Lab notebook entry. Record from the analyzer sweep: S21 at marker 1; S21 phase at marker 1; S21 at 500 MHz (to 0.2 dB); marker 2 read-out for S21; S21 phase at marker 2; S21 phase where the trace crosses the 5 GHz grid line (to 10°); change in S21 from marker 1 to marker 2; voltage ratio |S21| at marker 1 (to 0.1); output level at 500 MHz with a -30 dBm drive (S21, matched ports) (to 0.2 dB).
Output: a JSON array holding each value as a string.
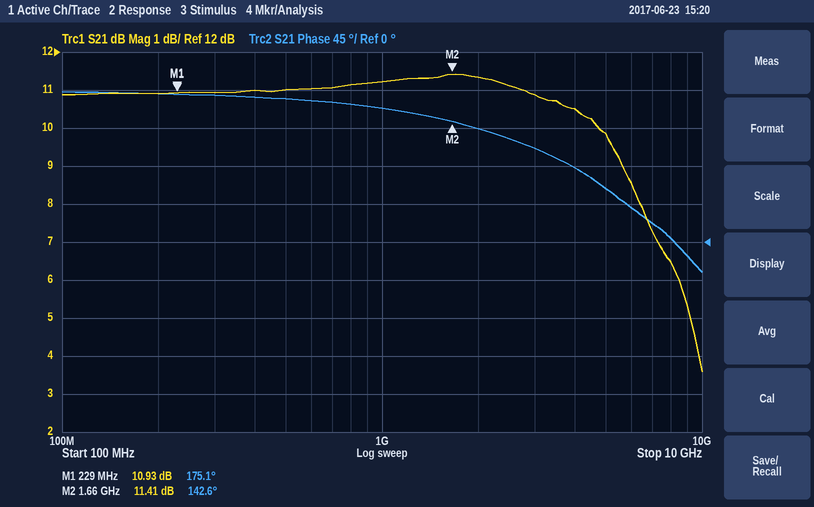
["10.93 dB", "175.1°", "11.0 dB", "11.41 dB", "142.6°", "60°", "0.48 dB", "3.5", "-19.0 dBm"]
